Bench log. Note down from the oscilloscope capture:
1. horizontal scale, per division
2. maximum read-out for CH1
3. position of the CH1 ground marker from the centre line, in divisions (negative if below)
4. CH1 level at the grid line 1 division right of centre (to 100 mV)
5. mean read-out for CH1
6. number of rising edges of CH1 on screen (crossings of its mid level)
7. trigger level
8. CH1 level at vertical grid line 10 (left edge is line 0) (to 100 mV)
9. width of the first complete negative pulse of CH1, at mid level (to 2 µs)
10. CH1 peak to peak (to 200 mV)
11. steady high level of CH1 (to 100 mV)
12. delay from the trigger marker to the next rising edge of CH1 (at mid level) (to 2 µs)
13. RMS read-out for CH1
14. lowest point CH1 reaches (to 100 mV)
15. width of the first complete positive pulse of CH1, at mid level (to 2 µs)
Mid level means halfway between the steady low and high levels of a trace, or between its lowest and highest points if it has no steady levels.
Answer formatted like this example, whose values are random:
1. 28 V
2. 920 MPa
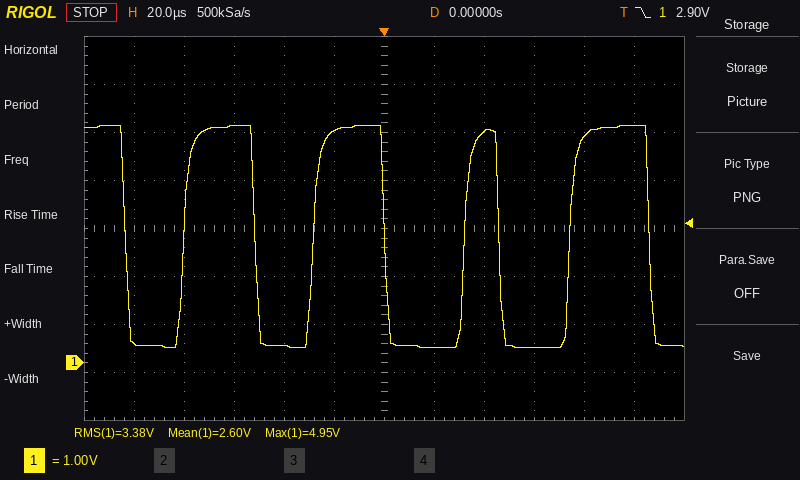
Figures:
1. 20 µs
2. 4.95 V
3. -2.8 div
4. 300 mV
5. 2.60 V
6. 4
7. 2.90 V
8. 4.7 V
9. 24 µs
10. 4.6 V
11. 4.9 V
12. 32 µs
13. 3.38 V
14. 300 mV
15. 28 µs
